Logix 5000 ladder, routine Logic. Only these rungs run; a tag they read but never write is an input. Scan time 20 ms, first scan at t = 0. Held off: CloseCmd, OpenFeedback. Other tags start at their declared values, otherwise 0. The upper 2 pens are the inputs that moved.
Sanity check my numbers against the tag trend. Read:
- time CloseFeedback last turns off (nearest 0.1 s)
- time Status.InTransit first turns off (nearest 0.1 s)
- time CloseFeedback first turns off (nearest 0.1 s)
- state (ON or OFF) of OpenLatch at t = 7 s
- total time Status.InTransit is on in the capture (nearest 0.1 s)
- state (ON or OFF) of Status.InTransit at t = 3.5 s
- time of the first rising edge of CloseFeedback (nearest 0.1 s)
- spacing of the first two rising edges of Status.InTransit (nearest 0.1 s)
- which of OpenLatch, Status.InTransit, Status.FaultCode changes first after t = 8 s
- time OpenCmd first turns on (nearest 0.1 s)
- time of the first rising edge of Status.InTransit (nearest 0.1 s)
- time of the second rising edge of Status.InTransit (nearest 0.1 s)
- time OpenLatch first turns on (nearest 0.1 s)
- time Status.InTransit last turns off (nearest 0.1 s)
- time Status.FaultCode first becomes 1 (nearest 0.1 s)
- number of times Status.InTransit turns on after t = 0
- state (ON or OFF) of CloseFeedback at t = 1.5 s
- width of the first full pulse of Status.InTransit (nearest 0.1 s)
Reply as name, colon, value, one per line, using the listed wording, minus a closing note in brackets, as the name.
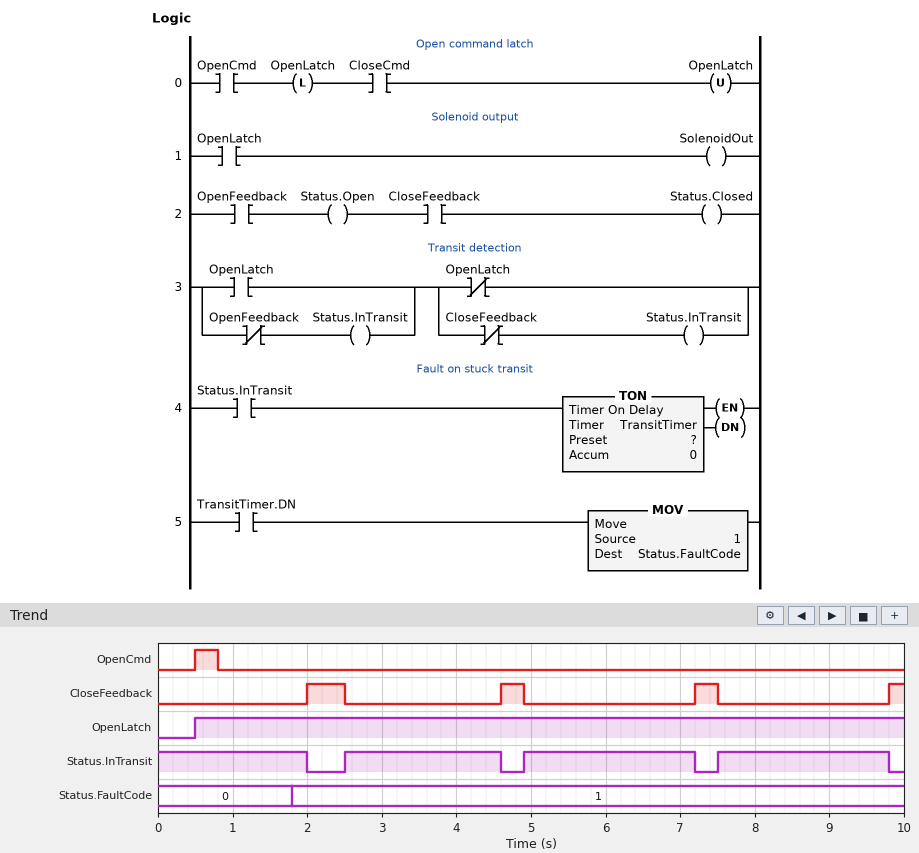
time CloseFeedback last turns off: 7.5 s
time Status.InTransit first turns off: 2.0 s
time CloseFeedback first turns off: 2.5 s
state (ON or OFF) of OpenLatch at t = 7 s: ON
total time Status.InTransit is on in the capture: 8.7 s
state (ON or OFF) of Status.InTransit at t = 3.5 s: ON
time of the first rising edge of CloseFeedback: 2.0 s
spacing of the first two rising edges of Status.InTransit: 2.4 s
which of OpenLatch, Status.InTransit, Status.FaultCode changes first after t = 8 s: Status.InTransit
time OpenCmd first turns on: 0.5 s
time of the first rising edge of Status.InTransit: 2.5 s
time of the second rising edge of Status.InTransit: 4.9 s
time OpenLatch first turns on: 0.5 s
time Status.InTransit last turns off: 9.8 s
time Status.FaultCode first becomes 1: 1.8 s
number of times Status.InTransit turns on after t = 0: 3
state (ON or OFF) of CloseFeedback at t = 1.5 s: OFF
width of the first full pulse of Status.InTransit: 2.1 s
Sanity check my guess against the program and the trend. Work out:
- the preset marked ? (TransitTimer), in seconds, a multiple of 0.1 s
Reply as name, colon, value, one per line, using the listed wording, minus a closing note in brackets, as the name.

the preset marked ? (TransitTimer), in seconds, a multiple of 0.1 s: 1.8 s
